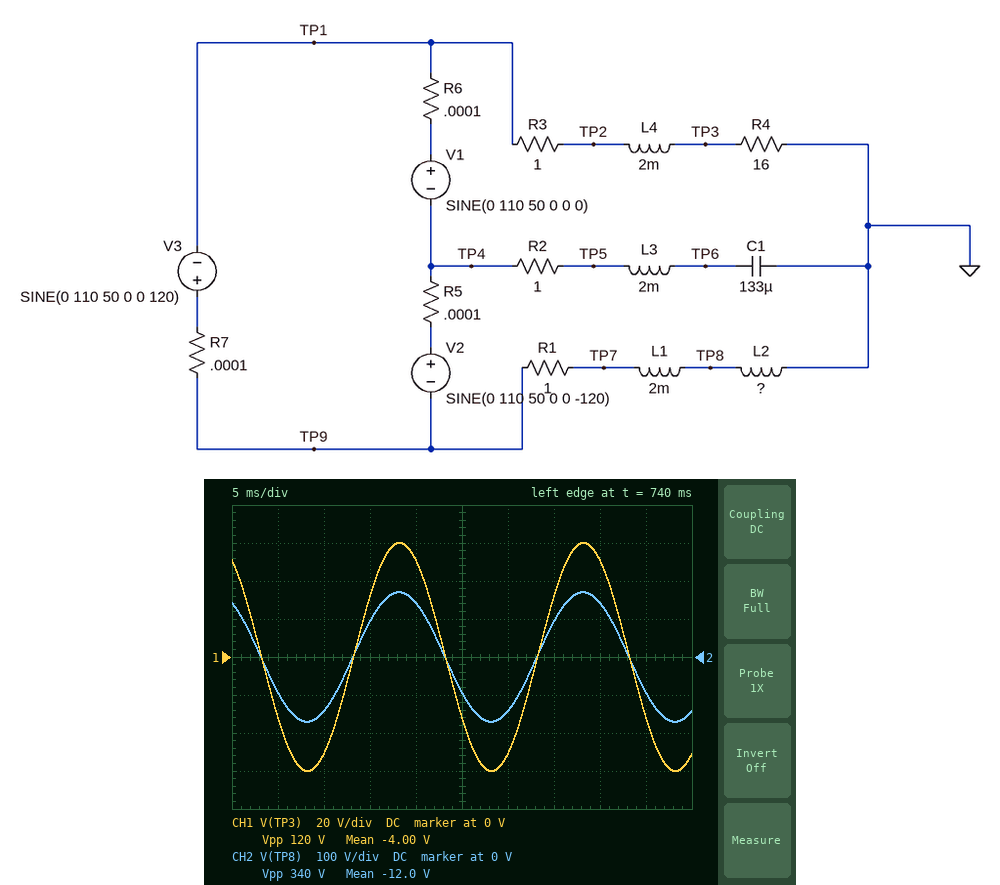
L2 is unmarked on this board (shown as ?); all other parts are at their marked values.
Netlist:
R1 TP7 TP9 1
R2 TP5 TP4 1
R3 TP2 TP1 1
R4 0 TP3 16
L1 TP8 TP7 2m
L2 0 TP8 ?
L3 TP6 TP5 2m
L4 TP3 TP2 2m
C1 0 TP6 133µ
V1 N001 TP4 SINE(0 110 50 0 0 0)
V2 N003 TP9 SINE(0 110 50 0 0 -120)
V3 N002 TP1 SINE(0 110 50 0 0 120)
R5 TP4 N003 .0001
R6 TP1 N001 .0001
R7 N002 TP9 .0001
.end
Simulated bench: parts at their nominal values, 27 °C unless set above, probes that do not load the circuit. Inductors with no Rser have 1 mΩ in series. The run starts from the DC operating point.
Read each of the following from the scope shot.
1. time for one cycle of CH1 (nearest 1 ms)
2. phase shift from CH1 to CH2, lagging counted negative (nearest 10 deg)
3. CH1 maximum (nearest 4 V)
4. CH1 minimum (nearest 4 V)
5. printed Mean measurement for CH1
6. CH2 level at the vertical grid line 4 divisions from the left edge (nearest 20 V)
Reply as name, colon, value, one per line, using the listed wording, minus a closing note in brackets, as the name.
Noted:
time for one cycle of CH1: 20 ms
phase shift from CH1 to CH2, lagging counted negative: 0 deg
CH1 maximum: 60 V
CH1 minimum: -60 V
printed Mean measurement for CH1: -4.00 V
CH2 level at the vertical grid line 4 divisions from the left edge: 140 V
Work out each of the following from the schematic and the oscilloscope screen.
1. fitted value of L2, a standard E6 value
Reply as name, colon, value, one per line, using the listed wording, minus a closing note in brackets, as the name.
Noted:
fitted value of L2, a standard E6 value: 100 mH
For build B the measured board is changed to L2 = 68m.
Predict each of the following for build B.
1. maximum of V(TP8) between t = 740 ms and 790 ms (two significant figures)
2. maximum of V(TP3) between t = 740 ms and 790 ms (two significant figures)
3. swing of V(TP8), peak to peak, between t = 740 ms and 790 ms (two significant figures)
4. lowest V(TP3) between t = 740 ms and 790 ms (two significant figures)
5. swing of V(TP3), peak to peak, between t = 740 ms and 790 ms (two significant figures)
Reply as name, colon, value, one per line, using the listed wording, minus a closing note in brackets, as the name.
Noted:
maximum of V(TP8) between t = 740 ms and 790 ms: 170 V
maximum of V(TP3) between t = 740 ms and 790 ms: 67 V
swing of V(TP8), peak to peak, between t = 740 ms and 790 ms: 330 V
lowest V(TP3) between t = 740 ms and 790 ms: -67 V
swing of V(TP3), peak to peak, between t = 740 ms and 790 ms: 130 V
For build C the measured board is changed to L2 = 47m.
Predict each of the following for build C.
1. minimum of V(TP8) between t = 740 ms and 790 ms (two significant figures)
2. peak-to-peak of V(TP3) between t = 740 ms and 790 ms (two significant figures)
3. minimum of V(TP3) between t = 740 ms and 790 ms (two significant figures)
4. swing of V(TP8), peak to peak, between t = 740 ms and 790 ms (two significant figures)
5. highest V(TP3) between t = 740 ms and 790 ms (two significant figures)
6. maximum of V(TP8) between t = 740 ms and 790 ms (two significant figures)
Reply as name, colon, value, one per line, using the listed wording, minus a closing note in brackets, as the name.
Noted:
minimum of V(TP8) between t = 740 ms and 790 ms: -150 V
peak-to-peak of V(TP3) between t = 740 ms and 790 ms: 160 V
minimum of V(TP3) between t = 740 ms and 790 ms: -79 V
swing of V(TP8), peak to peak, between t = 740 ms and 790 ms: 300 V
highest V(TP3) between t = 740 ms and 790 ms: 79 V
maximum of V(TP8) between t = 740 ms and 790 ms: 150 V
